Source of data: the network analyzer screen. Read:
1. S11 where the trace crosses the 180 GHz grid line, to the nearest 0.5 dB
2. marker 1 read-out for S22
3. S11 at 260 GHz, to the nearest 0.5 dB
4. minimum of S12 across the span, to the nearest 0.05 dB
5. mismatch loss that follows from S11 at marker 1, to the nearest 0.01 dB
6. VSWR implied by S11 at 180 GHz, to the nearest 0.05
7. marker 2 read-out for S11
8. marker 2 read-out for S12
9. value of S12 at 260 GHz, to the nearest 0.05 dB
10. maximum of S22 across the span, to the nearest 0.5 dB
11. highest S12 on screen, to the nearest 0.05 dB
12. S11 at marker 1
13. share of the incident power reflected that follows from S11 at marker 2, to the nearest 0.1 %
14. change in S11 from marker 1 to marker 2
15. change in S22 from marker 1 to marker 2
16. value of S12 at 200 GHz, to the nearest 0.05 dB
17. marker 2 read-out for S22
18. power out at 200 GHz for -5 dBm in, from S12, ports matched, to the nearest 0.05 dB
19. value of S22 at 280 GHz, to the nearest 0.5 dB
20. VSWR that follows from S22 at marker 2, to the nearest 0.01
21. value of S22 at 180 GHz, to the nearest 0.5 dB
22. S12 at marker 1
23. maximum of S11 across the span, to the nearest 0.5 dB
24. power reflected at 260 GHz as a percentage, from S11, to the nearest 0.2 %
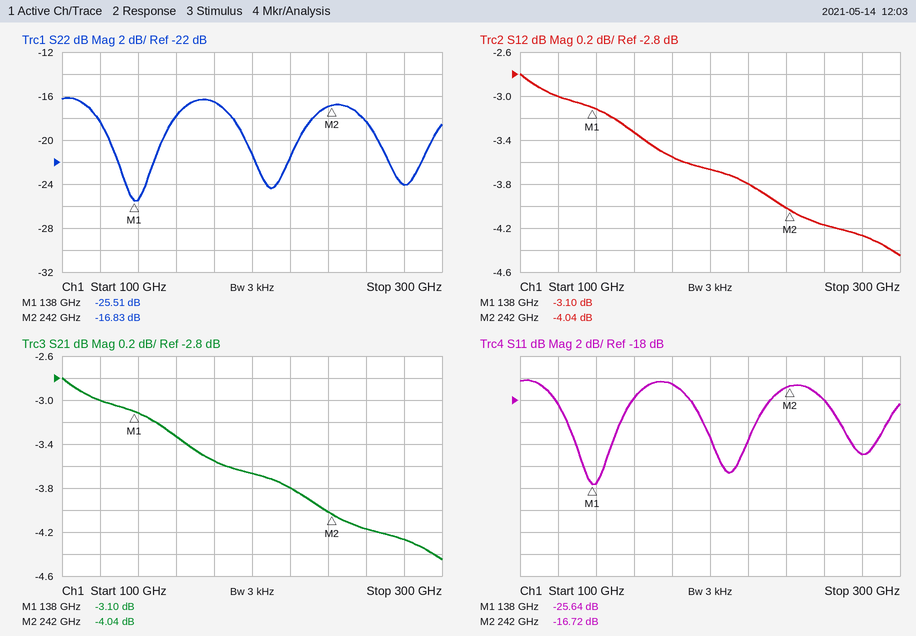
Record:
-16.5 dB
-25.51 dB
-18.0 dB
-4.45 dB
0.01 dB
1.35
-16.72 dB
-4.04 dB
-4.15 dB
-16.0 dB
-2.80 dB
-25.64 dB
2.1 %
8.92 dB
8.68 dB
-3.65 dB
-16.83 dB
-8.65 dBm
-24.0 dB
1.34
-16.5 dB
-3.10 dB
-16.0 dB
1.6 %
